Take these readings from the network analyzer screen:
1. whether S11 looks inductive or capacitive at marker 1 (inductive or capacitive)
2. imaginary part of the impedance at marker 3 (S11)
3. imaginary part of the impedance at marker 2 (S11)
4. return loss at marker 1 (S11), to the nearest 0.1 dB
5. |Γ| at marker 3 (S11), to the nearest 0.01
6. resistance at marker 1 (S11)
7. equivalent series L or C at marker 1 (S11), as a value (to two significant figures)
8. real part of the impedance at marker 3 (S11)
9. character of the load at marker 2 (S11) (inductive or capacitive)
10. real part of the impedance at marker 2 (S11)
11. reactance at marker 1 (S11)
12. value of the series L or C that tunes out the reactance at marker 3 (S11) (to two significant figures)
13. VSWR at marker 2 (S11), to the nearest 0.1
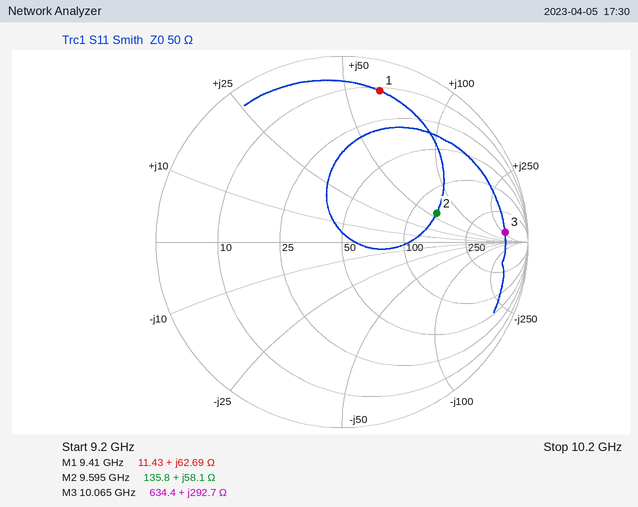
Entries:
inductive
+292.7 Ω
+58.1 Ω
1.5 dB
0.88
11.43 Ω
1.1 nH
634.4 Ω
inductive
135.8 Ω
+62.69 Ω
54 fF
3.3
